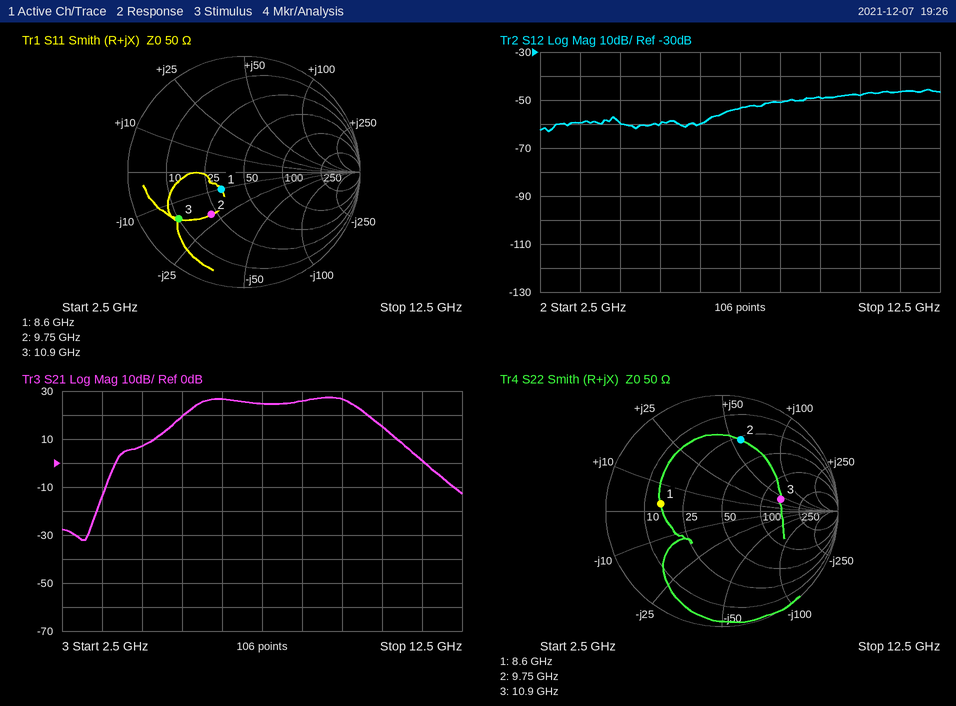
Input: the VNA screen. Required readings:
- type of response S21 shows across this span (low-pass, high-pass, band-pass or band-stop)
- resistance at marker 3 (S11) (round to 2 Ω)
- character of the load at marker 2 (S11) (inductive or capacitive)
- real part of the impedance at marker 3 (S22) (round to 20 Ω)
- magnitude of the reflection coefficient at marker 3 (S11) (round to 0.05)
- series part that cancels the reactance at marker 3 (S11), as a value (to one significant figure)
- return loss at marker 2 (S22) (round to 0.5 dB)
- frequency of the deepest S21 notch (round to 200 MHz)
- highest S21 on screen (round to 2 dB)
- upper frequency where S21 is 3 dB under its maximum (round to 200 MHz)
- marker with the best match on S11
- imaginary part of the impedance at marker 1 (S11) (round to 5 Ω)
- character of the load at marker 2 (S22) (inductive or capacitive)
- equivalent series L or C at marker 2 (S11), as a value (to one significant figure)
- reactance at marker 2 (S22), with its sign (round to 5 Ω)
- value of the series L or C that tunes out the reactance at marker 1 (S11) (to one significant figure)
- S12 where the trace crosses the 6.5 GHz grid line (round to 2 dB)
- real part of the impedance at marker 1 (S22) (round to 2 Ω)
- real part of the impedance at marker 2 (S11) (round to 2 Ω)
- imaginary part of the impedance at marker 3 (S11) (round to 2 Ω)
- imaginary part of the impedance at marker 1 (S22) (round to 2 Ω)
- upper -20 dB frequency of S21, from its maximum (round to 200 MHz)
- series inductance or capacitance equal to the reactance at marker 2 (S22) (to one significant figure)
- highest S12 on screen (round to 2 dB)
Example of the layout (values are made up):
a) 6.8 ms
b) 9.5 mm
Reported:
a) band-pass
b) 10 Ω
c) capacitive
d) 140 Ω
e) 0.70
f) 200 pH
g) 4.0 dB
h) 3.0 GHz
i) 28 dB
j) 9.8 GHz
k) marker 1
l) -10 Ω
m) inductive
n) 800 fF
o) +55 Ω
p) 200 pH
q) -60 dB
r) 16 Ω
s) 22 Ω
t) -16 Ω
u) +2 Ω
v) 11.0 GHz
w) 900 pH
x) -46 dB
